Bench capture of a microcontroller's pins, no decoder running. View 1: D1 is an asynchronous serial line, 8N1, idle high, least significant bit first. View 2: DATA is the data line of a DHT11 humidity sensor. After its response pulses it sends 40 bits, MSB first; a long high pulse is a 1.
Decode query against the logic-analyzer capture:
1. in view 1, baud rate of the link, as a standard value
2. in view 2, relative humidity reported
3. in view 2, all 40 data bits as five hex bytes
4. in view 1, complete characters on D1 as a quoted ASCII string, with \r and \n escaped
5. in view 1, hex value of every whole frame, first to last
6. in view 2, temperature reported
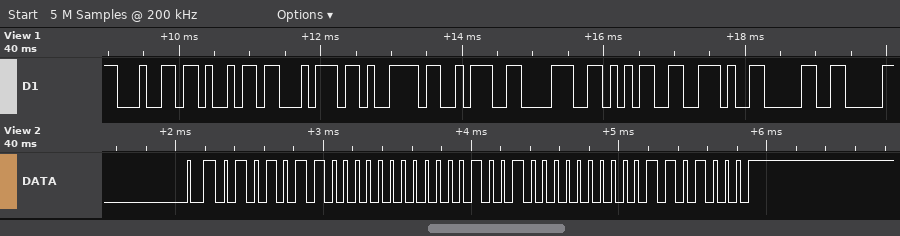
9600 baud
86 %
56 00 12 00 68
"dity:85.0"
0x64 0x69 0x74 0x79 0x3A 0x38 0x35 0x2E 0x30
18.0 °C
